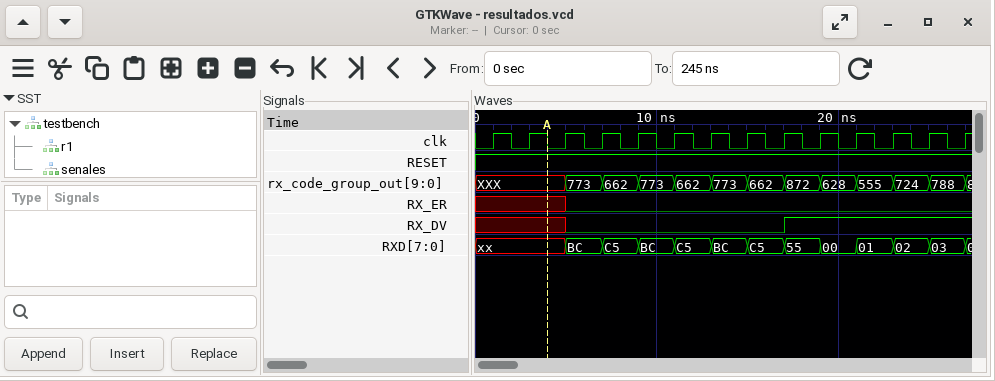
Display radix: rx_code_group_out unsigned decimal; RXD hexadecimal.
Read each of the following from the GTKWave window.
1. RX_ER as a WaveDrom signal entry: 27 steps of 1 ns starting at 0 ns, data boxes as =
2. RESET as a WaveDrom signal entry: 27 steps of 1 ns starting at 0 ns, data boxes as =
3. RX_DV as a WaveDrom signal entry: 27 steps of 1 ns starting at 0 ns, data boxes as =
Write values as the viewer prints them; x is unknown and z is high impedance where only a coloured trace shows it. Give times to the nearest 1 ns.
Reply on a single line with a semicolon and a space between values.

{name: 'RX_ER', wave: 'x....0.....................'}; {name: 'RESET', wave: '1..........................'}; {name: 'RX_DV', wave: 'x....0...........1.........'}
